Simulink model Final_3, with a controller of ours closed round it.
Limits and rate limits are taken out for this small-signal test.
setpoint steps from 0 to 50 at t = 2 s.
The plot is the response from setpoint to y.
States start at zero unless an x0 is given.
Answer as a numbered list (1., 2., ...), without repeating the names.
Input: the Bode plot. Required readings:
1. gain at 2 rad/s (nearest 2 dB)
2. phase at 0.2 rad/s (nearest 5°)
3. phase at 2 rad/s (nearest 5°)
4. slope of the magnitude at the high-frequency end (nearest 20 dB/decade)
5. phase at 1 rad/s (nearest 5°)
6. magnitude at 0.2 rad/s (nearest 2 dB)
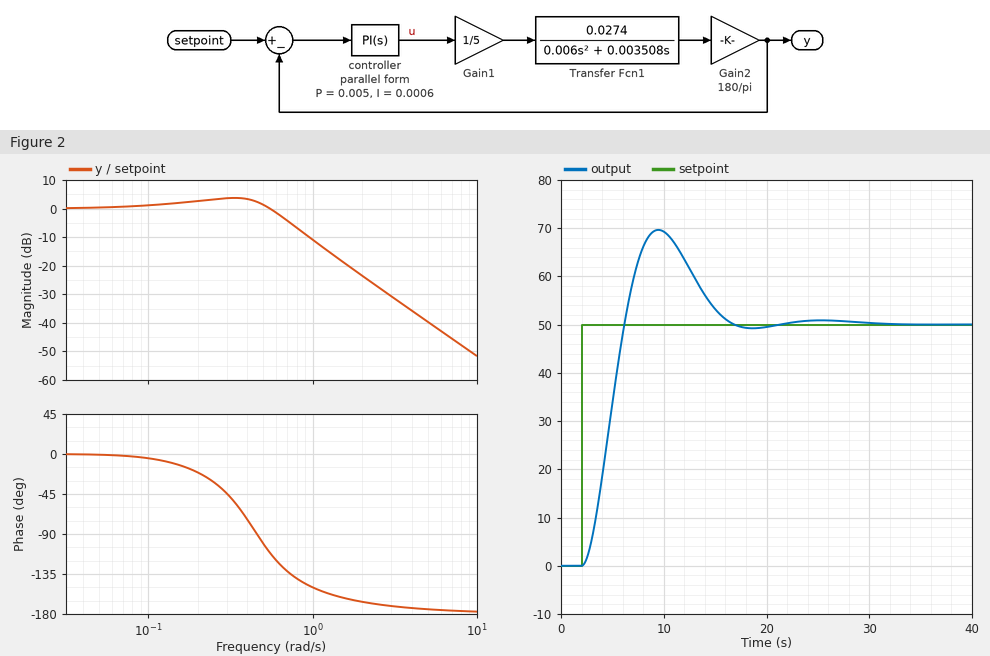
1. -24 dB
2. -20°
3. -165°
4. -40 dB/decade
5. -150°
6. 2 dB
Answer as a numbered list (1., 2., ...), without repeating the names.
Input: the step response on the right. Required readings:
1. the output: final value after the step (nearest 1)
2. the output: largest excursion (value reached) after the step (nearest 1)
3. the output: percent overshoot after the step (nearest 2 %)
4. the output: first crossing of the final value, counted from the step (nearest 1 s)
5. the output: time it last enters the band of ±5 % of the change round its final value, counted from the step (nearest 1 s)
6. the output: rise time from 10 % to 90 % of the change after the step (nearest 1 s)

1. 50
2. 70
3. 40 %
4. 4 s
5. 13 s
6. 3 s
